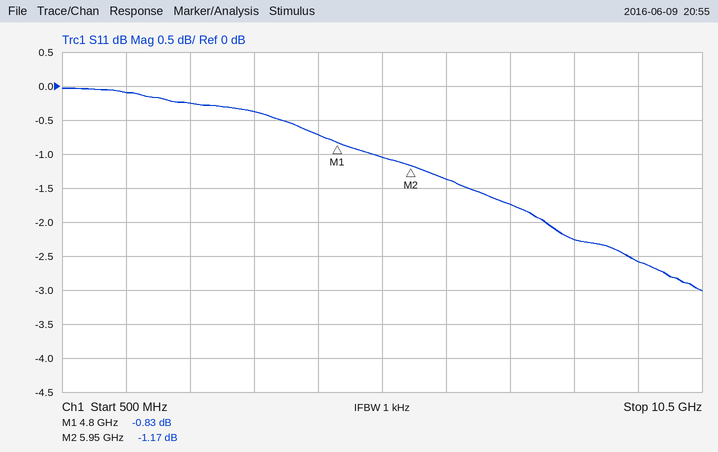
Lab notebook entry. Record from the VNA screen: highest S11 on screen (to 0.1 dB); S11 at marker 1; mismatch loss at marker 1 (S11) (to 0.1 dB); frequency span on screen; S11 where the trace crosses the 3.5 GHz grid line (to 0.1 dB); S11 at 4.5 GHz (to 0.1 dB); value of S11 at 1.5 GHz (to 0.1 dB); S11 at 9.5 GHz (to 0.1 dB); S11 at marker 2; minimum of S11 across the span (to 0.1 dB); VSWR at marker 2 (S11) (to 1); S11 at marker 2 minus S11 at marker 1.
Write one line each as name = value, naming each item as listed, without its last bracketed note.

highest S11 on screen = 0.0 dB
S11 at marker 1 = -0.83 dB
mismatch loss at marker 1 (S11) = 7.6 dB
frequency span on screen = 10 GHz
S11 where the trace crosses the 3.5 GHz grid line = -0.4 dB
S11 at 4.5 GHz = -0.7 dB
value of S11 at 1.5 GHz = -0.1 dB
S11 at 9.5 GHz = -2.6 dB
S11 at marker 2 = -1.17 dB
minimum of S11 across the span = -3.0 dB
VSWR at marker 2 (S11) = 15
S11 at marker 2 minus S11 at marker 1 = -0.34 dB
